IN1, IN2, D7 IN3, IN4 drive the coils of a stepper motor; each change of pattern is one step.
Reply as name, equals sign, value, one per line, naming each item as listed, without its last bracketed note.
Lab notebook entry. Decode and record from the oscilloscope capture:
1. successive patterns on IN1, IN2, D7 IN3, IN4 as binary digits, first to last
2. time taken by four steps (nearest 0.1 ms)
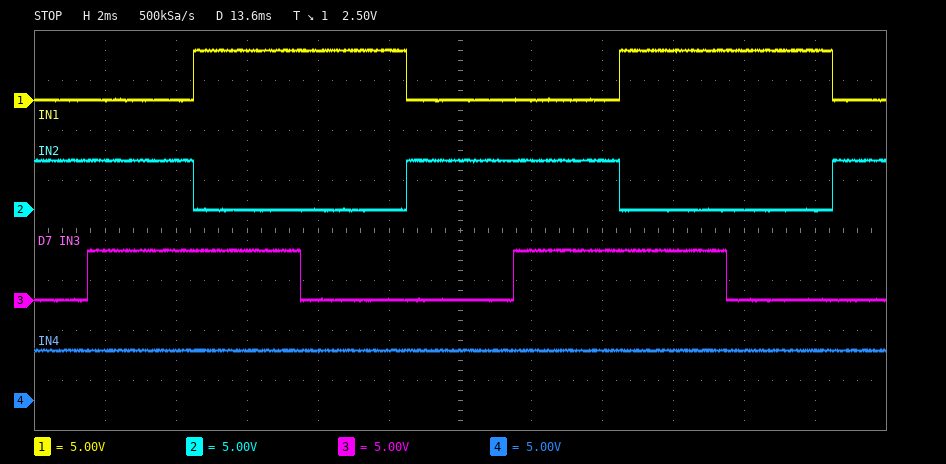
successive patterns on IN1, IN2, D7 IN3, IN4 as binary digits, first to last = 0101 0111 1011 1001 0101 0111 1011 1001 0101
time taken by four steps = 12.0 ms
